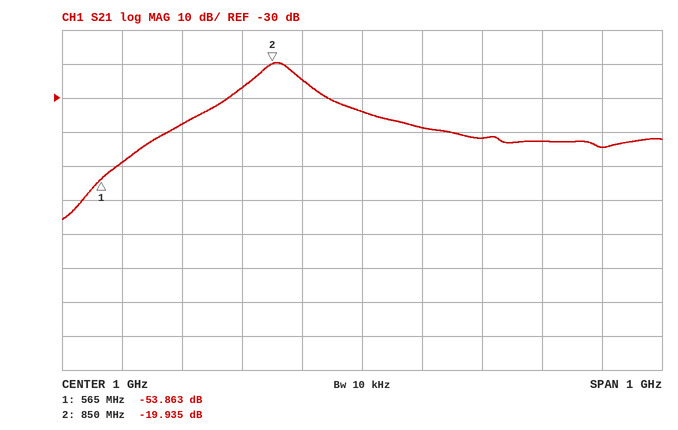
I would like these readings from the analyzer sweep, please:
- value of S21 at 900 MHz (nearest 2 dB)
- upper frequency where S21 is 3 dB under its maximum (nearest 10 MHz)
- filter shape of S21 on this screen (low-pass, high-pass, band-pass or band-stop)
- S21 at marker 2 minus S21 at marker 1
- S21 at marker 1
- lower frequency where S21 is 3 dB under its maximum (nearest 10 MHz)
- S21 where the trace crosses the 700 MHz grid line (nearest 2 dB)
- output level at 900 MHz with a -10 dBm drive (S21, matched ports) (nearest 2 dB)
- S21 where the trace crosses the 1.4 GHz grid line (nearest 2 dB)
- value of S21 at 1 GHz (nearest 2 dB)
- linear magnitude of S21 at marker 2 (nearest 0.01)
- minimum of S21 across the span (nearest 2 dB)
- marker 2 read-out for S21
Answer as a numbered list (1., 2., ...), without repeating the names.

1. -24 dB
2. 890 MHz
3. band-pass
4. 33.928 dB
5. -53.863 dB
6. 830 MHz
7. -38 dB
8. -34 dBm
9. -44 dB
10. -34 dB
11. 0.10
12. -66 dB
13. -19.935 dB
